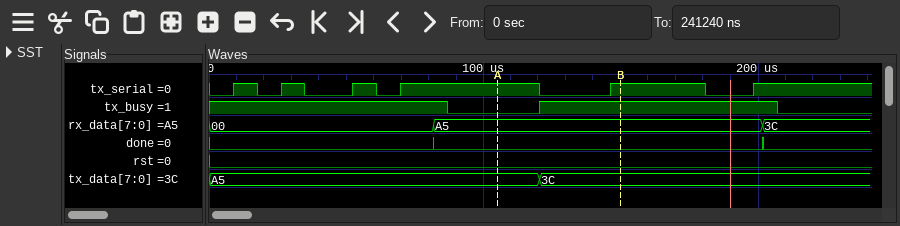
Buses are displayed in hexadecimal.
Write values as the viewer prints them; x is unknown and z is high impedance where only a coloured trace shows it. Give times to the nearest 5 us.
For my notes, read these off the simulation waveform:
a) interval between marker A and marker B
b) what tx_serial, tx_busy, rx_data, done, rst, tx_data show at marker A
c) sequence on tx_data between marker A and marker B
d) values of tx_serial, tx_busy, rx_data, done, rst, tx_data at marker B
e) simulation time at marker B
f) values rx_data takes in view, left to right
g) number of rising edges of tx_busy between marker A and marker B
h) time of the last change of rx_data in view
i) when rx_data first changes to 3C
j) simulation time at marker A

45 us
tx_serial=1, tx_busy=0, rx_data=A5, done=0, rst=0, tx_data=A5
A5, 3C
tx_serial=1, tx_busy=1, rx_data=A5, done=0, rst=0, tx_data=3C
150 us
00, A5, 3C
1
200 us
200 us
105 us
